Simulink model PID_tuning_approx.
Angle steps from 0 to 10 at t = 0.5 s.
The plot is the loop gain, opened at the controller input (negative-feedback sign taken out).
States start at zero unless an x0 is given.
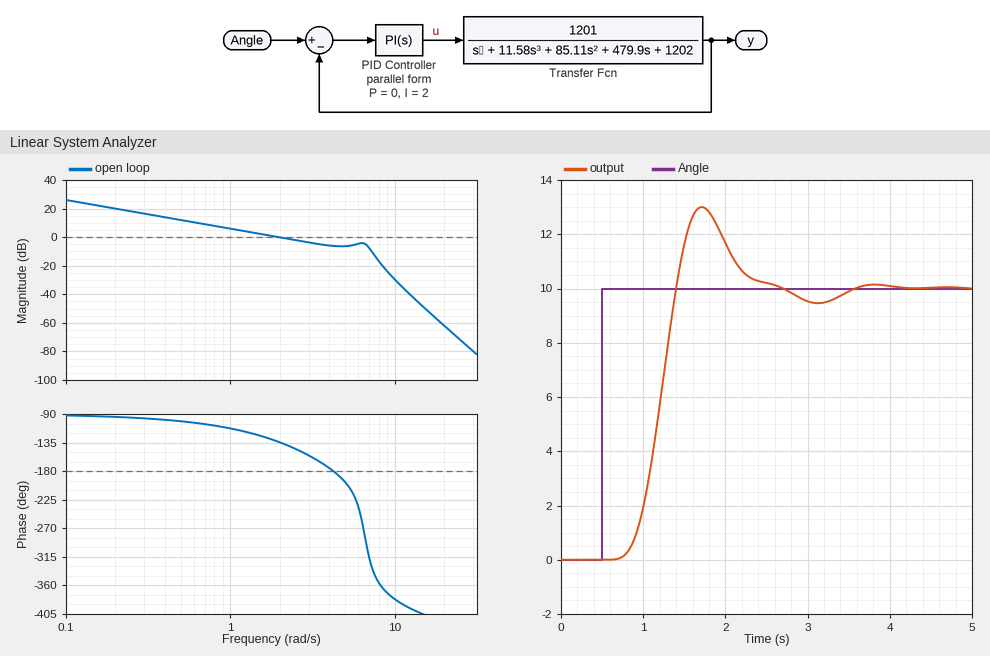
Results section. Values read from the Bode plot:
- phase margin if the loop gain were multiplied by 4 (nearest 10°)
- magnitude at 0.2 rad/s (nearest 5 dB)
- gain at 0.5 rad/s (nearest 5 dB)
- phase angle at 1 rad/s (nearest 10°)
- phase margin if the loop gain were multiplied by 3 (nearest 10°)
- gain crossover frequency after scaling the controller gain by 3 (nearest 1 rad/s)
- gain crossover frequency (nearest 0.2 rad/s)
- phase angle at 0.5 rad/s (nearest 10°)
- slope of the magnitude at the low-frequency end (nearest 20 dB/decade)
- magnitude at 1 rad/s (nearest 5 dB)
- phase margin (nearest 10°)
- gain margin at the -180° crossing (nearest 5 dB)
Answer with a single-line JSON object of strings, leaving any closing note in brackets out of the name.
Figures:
{"phase margin if the loop gain were multiplied by 4": "-160°", "magnitude at 0.2 rad/s": "20 dB", "gain at 0.5 rad/s": "10 dB", "phase angle at 1 rad/s": "-110°", "phase margin if the loop gain were multiplied by 3": "-150°", "gain crossover frequency after scaling the controller gain by 3": "7 rad/s", "gain crossover frequency": "2.0 rad/s", "phase angle at 0.5 rad/s": "-100°", "slope of the magnitude at the low-frequency end": "-20 dB/decade", "magnitude at 1 rad/s": "5 dB", "phase margin": "50°", "gain margin at the -180° crossing": "5 dB"}
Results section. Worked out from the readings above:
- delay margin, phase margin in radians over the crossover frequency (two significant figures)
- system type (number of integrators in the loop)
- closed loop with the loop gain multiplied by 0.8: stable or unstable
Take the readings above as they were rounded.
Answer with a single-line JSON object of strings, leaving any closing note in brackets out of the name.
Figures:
{"delay margin, phase margin in radians over the crossover frequency": "0.44 s", "system type": "1", "closed loop with the loop gain multiplied by 0.8: stable or unstable": "stable"}
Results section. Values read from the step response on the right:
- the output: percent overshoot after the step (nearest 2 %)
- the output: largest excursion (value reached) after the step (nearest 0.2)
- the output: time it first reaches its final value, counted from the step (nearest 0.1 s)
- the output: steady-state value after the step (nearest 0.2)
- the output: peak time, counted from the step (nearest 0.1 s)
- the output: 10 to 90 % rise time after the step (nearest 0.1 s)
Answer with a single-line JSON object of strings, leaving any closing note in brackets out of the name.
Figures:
{"the output: percent overshoot after the step": "30 %", "the output: largest excursion (value reached) after the step": "13.0", "the output: time it first reaches its final value, counted from the step": "0.9 s", "the output: steady-state value after the step": "10.0", "the output: peak time, counted from the step": "1.2 s", "the output: 10 to 90 % rise time after the step": "0.4 s"}
